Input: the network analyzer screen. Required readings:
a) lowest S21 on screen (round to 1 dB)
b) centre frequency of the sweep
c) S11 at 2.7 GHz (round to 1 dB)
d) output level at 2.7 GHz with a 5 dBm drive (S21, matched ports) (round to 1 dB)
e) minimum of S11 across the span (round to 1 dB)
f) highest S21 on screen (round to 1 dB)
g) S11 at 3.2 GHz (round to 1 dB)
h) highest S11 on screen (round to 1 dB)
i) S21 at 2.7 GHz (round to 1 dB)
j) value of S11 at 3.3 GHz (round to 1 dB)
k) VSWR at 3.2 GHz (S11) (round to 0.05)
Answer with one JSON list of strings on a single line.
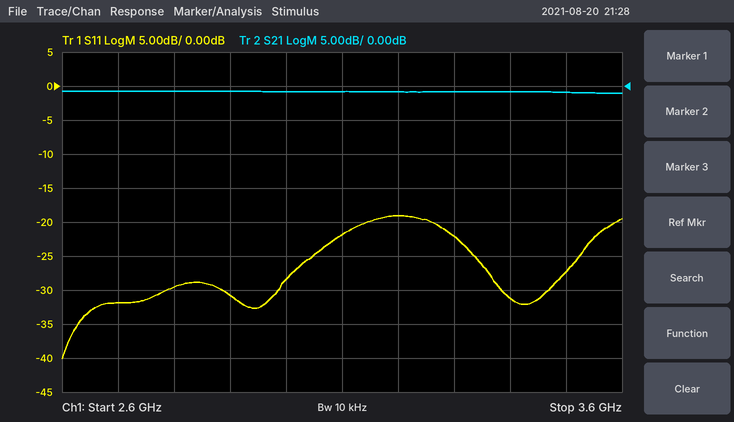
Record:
["-1 dB", "3.1 GHz", "-32 dB", "4 dBm", "-40 dB", "-1 dB", "-19 dB", "-19 dB", "-1 dB", "-22 dB", "1.25"]
